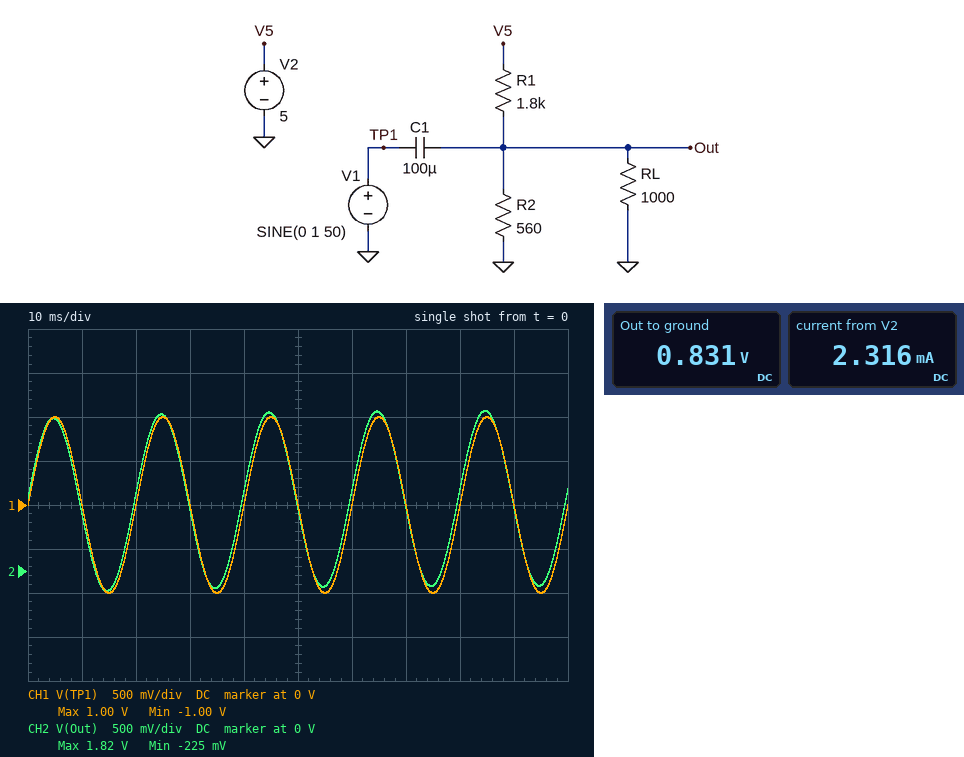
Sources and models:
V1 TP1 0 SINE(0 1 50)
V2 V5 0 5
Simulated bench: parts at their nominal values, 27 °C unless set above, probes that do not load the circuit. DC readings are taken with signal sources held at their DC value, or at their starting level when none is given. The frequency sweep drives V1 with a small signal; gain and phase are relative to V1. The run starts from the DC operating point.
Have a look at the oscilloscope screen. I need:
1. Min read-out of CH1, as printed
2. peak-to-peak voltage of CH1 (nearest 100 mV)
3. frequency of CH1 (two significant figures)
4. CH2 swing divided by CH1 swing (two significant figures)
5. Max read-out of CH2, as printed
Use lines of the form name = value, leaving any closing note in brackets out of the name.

Min read-out of CH1, as printed = -1.00 V
peak-to-peak voltage of CH1 = 2.0 V
frequency of CH1 = 50 Hz
CH2 swing divided by CH1 swing = 1.0
Max read-out of CH2, as printed = 1.82 V
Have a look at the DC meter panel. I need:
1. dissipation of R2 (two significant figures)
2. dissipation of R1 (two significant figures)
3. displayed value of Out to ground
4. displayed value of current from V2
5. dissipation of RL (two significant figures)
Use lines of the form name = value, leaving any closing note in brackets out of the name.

dissipation of R2 = 1.2 mW
dissipation of R1 = 9.7 mW
displayed value of Out to ground = 0.831 V
displayed value of current from V2 = 2.316 mA
dissipation of RL = 690 µW
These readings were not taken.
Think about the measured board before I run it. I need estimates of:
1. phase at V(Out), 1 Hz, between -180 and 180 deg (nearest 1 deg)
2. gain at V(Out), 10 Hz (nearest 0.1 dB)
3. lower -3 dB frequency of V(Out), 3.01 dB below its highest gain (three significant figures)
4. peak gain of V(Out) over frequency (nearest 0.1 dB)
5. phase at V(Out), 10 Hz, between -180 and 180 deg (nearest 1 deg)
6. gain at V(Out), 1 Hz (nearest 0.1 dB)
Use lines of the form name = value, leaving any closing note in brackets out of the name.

phase at V(Out), 1 Hz, between -180 and 180 deg = 79 deg
gain at V(Out), 10 Hz = -1.1 dB
lower -3 dB frequency of V(Out), 3.01 dB below its highest gain = 5.32 Hz
peak gain of V(Out) over frequency = 0 dB
phase at V(Out), 10 Hz, between -180 and 180 deg = 28 deg
gain at V(Out), 1 Hz = -14.7 dB
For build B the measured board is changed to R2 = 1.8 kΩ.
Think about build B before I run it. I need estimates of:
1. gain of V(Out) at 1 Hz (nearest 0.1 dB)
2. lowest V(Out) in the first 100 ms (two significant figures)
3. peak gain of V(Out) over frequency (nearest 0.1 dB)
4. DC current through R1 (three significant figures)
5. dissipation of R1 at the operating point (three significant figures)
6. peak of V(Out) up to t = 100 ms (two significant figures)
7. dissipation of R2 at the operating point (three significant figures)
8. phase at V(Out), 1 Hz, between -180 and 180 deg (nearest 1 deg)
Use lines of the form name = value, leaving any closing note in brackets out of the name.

gain of V(Out) at 1 Hz = -10.9 dB
lowest V(Out) in the first 100 ms = 270 mV
peak gain of V(Out) over frequency = 0 dB
DC current through R1 = 2.05 mA
dissipation of R1 at the operating point = 7.54 mW
peak of V(Out) up to t = 100 ms = 2.3 V
dissipation of R2 at the operating point = 962 µW
phase at V(Out), 1 Hz, between -180 and 180 deg = 73 deg
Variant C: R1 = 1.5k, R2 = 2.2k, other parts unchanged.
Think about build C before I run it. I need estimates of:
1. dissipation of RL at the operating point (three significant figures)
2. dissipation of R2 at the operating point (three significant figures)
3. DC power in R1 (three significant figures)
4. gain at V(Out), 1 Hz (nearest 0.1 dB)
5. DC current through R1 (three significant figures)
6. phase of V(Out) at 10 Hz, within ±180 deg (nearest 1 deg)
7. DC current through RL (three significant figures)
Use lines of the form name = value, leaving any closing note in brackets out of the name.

dissipation of RL at the operating point = 2.47 mW
dissipation of R2 at the operating point = 1.12 mW
DC power in R1 = 7.84 mW
gain at V(Out), 1 Hz = -10.9 dB
DC current through R1 = 2.29 mA
phase of V(Out) at 10 Hz, within ±180 deg = 19 deg
DC current through RL = 1.57 mA
